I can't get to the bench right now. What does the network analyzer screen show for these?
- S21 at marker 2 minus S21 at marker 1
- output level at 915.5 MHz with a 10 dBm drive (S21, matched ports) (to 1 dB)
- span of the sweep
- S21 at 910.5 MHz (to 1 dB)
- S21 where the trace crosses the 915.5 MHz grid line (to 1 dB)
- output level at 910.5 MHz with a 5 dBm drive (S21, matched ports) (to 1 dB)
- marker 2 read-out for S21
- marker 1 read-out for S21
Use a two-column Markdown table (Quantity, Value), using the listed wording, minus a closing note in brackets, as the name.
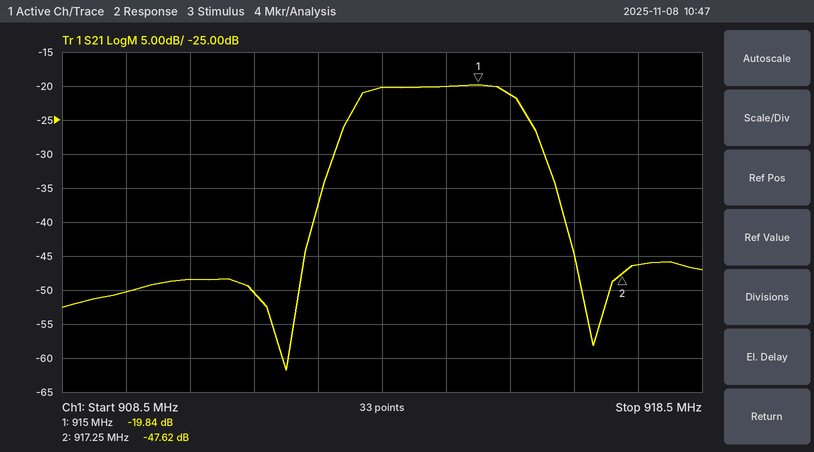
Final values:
| Quantity | Value |
|---|---|
| S21 at marker 2 minus S21 at marker 1 | -27.78 dB |
| output level at 915.5 MHz with a 10 dBm drive (S21, matched ports) | -11 dBm |
| span of the sweep | 10 MHz |
| S21 at 910.5 MHz | -48 dB |
| S21 where the trace crosses the 915.5 MHz grid line | -21 dB |
| output level at 910.5 MHz with a 5 dBm drive (S21, matched ports) | -43 dBm |
| marker 2 read-out for S21 | -47.62 dB |
| marker 1 read-out for S21 | -19.84 dB |
